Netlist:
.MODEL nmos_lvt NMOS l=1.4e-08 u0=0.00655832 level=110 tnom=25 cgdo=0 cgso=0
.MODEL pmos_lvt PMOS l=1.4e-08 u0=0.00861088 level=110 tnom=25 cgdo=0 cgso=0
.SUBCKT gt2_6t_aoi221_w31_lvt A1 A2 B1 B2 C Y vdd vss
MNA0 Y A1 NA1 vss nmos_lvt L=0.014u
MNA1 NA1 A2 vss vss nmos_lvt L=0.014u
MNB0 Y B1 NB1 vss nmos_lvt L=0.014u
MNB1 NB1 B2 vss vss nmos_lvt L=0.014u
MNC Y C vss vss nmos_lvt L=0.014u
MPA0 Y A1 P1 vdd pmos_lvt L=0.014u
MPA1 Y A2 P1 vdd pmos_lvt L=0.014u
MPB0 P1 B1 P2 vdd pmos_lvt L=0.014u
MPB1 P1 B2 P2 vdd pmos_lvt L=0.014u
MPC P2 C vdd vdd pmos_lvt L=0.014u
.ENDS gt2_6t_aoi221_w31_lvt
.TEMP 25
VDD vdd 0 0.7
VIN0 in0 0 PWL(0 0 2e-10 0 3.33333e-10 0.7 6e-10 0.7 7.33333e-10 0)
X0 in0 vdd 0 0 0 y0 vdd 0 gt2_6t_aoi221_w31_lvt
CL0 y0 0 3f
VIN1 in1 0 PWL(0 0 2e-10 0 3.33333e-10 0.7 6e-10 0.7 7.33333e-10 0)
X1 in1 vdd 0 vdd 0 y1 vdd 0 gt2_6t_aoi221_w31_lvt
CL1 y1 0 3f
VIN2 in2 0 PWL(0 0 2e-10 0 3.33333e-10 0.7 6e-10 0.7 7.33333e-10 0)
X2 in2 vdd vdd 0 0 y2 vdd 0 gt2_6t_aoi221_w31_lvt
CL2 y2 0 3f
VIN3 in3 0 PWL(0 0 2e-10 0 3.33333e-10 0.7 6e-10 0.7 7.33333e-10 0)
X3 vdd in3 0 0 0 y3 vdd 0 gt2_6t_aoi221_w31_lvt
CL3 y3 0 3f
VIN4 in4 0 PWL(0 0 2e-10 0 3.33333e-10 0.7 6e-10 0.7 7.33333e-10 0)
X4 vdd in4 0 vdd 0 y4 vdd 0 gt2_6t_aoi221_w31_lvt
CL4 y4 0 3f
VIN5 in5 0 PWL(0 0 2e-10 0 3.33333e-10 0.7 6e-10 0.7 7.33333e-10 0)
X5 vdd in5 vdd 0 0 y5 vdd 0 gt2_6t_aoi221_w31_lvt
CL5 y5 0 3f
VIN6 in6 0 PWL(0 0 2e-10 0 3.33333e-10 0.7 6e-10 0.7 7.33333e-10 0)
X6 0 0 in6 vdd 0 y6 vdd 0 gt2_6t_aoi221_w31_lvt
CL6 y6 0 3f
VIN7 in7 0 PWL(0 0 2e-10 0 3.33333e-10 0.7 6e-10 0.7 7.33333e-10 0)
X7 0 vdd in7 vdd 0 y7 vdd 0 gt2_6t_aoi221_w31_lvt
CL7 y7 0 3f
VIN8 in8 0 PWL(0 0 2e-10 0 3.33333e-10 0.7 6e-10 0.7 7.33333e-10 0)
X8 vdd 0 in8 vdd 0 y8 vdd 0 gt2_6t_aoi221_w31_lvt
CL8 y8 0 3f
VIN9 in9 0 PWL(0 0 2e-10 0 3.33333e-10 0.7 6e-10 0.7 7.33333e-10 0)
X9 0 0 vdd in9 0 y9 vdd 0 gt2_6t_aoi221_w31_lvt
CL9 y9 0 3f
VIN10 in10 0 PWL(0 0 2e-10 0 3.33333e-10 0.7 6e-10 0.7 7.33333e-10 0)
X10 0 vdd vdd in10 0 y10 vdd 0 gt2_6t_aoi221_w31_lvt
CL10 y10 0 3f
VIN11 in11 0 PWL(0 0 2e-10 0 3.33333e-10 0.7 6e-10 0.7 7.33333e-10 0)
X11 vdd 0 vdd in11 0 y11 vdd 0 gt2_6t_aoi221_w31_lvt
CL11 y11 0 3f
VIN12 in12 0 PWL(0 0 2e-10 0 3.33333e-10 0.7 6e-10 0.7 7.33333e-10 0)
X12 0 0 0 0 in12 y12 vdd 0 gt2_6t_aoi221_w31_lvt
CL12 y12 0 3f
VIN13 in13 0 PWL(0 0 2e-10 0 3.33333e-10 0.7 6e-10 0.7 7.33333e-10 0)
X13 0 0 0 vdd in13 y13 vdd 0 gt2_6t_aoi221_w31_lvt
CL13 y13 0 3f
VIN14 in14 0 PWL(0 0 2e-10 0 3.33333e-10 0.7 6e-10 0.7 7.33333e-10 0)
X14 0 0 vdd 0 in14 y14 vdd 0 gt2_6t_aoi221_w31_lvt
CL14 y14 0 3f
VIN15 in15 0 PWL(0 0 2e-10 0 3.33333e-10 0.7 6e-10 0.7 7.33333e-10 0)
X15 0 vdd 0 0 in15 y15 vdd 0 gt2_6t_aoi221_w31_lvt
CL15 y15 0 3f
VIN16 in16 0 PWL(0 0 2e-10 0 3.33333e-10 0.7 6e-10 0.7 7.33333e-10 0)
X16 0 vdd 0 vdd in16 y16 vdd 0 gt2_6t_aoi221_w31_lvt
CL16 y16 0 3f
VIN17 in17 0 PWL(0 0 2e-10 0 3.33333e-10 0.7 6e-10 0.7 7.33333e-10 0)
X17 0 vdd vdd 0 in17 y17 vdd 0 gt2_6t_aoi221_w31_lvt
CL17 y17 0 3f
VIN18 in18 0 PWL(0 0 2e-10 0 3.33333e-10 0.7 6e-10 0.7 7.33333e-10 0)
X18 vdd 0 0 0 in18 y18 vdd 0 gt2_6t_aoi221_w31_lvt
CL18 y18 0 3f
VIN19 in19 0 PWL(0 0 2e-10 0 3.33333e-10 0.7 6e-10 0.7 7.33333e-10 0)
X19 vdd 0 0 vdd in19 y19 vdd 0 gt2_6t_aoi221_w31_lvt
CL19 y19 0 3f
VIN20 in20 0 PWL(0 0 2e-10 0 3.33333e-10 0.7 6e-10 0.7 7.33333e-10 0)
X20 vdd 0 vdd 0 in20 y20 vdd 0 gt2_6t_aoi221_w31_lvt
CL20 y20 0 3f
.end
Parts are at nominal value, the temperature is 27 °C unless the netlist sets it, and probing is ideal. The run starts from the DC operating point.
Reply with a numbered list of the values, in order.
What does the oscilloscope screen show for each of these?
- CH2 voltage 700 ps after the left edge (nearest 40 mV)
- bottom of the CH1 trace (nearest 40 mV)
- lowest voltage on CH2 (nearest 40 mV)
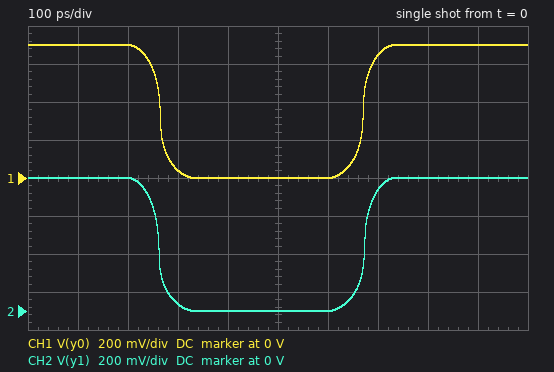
1. 640 mV
2. 0 V
3. 0 V
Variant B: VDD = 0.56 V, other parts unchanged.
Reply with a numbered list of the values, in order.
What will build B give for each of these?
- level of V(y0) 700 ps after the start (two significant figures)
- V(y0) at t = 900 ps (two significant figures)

1. 490 mV
2. 560 mV
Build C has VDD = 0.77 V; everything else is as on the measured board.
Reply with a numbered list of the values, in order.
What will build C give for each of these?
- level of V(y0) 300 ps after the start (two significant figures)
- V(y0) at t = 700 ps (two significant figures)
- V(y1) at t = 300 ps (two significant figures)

1. 71 mV
2. 720 mV
3. 64 mV
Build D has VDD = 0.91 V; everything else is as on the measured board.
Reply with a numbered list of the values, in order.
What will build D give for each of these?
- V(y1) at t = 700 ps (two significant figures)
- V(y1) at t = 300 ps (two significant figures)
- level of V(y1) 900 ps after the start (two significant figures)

1. 860 mV
2. 140 mV
3. 910 mV
